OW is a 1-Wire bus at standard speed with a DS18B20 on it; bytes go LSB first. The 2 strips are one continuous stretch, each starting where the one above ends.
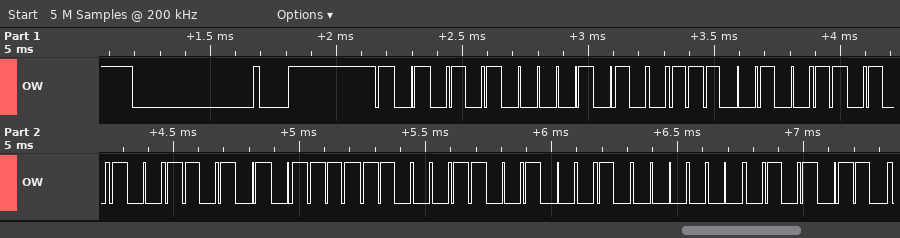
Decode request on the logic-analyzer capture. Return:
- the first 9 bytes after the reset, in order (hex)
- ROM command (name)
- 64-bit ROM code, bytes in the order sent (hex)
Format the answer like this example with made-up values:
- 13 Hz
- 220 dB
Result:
- 55 28 27 2B AB 1F 13 01 6A
- Match ROM
- 28 27 2B AB 1F 13 01 6A
